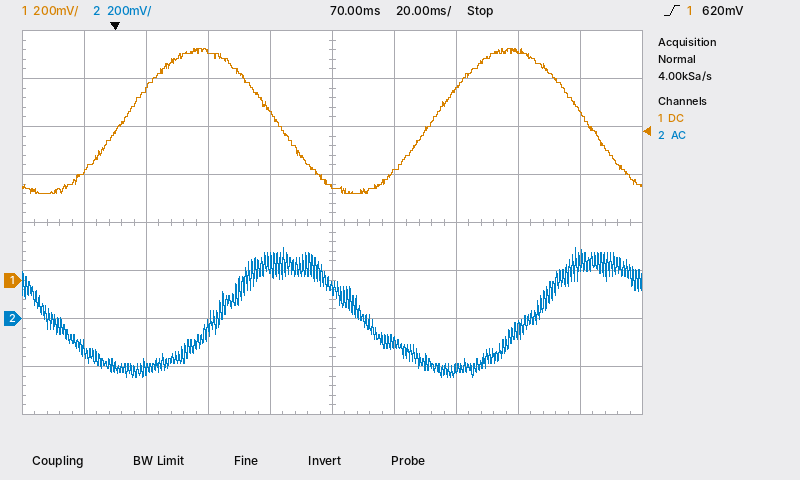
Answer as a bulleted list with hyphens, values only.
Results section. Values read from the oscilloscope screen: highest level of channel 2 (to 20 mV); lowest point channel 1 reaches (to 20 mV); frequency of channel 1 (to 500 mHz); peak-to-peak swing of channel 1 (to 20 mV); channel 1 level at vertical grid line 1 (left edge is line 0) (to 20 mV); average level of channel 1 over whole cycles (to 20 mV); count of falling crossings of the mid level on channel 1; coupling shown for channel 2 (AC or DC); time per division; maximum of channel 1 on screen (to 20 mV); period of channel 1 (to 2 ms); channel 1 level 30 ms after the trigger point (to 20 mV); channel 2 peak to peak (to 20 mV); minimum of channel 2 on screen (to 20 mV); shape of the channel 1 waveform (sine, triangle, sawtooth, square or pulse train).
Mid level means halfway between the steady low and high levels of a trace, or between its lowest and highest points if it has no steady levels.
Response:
- 300 mV
- 360 mV
- 10.0 Hz
- 600 mV
- 460 mV
- 660 mV
- 2
- AC
- 20 ms
- 960 mV
- 100 ms
- 960 mV
- 540 mV
- -240 mV
- sine
